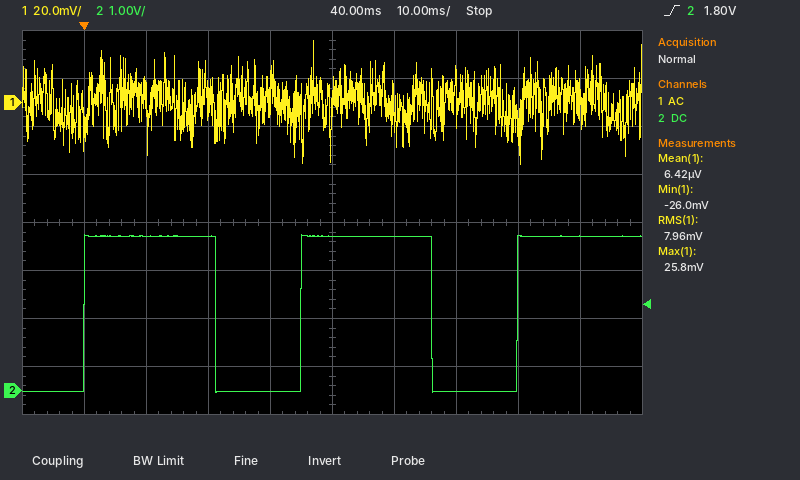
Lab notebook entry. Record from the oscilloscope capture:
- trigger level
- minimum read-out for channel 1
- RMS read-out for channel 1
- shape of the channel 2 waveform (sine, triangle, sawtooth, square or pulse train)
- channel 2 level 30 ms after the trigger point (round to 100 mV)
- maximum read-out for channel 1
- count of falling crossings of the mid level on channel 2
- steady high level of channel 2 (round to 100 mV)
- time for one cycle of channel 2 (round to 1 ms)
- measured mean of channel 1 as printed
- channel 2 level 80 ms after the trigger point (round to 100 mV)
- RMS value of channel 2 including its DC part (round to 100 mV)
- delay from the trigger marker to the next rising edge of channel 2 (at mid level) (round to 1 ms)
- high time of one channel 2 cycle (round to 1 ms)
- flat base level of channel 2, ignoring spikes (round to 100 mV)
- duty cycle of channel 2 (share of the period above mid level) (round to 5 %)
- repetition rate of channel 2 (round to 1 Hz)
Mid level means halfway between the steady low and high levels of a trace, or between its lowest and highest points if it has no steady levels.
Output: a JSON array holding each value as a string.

["1.80 V", "-26.0 mV", "7.96 mV", "pulse train", "0.0 V", "25.8 mV", "2", "3.2 V", "35 ms", "6.42 µV", "3.2 V", "2.5 V", "35 ms", "21 ms", "0.0 V", "60 %", "29 Hz"]
